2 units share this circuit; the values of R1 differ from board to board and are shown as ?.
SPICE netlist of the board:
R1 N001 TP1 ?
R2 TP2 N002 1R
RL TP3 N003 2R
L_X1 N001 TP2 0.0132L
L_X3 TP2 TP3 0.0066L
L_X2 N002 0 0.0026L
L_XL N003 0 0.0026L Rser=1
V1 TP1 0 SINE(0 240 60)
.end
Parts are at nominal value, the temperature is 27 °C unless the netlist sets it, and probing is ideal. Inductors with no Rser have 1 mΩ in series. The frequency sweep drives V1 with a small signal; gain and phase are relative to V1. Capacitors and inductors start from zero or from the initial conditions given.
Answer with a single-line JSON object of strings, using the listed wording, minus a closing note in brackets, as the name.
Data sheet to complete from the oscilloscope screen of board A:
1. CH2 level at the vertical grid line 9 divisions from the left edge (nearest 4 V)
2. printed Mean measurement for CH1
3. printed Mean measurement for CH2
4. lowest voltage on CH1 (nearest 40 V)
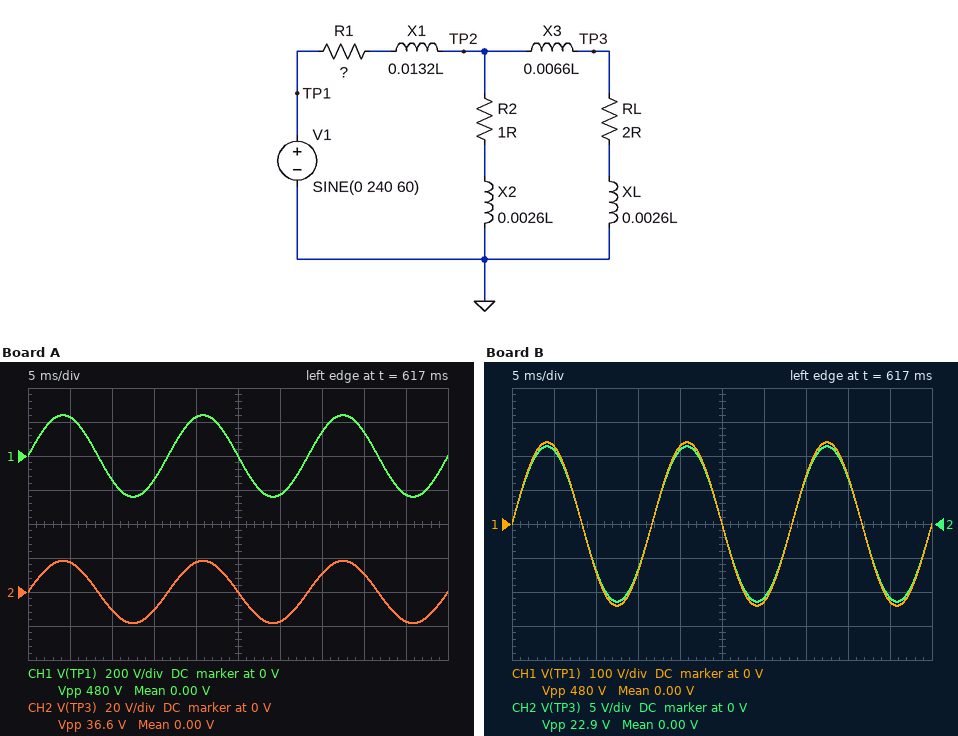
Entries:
{"CH2 level at the vertical grid line 9 divisions from the left edge": "-16 V", "printed Mean measurement for CH1": "0.00 V", "printed Mean measurement for CH2": "0.00 V", "lowest voltage on CH1": "-240 V"}
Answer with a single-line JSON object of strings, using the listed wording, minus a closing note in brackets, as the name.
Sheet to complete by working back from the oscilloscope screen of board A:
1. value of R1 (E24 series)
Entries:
{"value of R1": "9.1 Ω"}
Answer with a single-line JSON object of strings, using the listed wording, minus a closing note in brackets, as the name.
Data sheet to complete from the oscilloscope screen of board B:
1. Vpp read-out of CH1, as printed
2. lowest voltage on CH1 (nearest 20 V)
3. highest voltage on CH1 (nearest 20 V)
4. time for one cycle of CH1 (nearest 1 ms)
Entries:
{"Vpp read-out of CH1, as printed": "480 V", "lowest voltage on CH1": "-240 V", "highest voltage on CH1": "240 V", "time for one cycle of CH1": "17 ms"}
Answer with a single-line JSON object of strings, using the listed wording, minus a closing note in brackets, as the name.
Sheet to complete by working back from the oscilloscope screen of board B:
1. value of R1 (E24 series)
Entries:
{"value of R1": "15 Ω"}
